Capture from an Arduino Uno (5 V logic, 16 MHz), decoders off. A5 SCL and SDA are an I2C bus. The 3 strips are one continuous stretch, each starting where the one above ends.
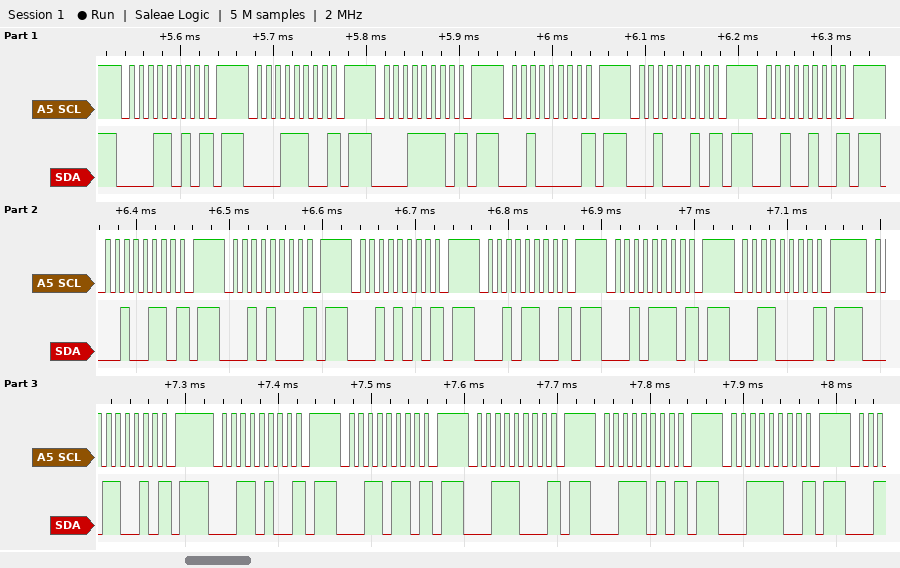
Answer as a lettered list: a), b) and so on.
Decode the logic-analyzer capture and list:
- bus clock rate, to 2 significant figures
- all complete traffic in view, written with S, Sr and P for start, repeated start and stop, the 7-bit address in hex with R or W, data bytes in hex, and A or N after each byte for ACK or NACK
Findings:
a) 100 kHz
b) S 0DW N P S 0EW N P S 0FW N P S 10W N P S 11W N P S 12W N P S 13W N P S 14W N P S 15W N P S 16W N P S 17W N P S 18W N P S 19W N P S 1AW N P S 1BW N P S 1CW N P S 1DW N P S 1EW N P
